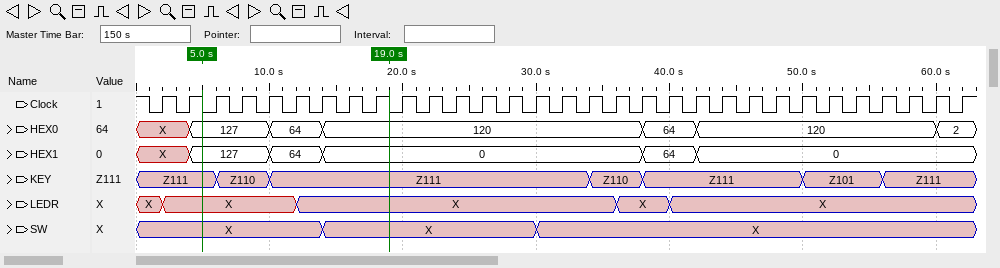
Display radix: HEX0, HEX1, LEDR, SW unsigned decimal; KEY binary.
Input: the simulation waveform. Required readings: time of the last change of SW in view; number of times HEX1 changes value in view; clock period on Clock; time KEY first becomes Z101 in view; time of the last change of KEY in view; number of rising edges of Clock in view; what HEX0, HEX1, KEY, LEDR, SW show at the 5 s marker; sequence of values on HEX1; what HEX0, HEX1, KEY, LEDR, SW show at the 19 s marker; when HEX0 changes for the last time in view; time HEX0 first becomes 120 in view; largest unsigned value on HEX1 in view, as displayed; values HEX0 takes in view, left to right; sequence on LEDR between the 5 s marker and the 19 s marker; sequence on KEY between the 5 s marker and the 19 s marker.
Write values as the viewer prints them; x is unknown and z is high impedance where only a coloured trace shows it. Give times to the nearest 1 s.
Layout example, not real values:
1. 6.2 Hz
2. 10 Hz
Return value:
1. 30 s
2. 5
3. 2 s
4. 50 s
5. 56 s
6. 31
7. HEX0=127, HEX1=127, KEY=Z111, LEDR=X, SW=X
8. X, 127, 64, 0, 64, 0
9. HEX0=120, HEX1=0, KEY=Z111, LEDR=X, SW=X
10. 60 s
11. 14 s
12. 127
13. X, 127, 64, 120, 64, 120, 2
14. X, X
15. Z111, Z110, Z111
